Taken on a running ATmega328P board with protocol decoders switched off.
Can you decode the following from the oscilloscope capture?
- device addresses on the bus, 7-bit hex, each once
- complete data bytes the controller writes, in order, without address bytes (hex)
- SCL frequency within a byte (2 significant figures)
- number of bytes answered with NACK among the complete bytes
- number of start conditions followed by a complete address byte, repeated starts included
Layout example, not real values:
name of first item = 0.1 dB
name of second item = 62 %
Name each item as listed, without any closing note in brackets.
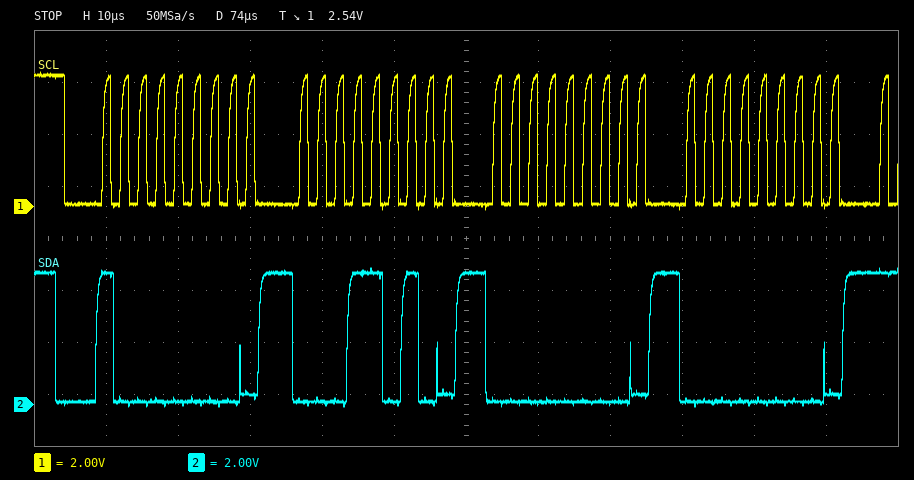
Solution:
device addresses on the bus, 7-bit hex, each once = 0x40
complete data bytes the controller writes, in order, without address bytes = 1A 00 00
SCL frequency within a byte = 400 kHz
number of bytes answered with NACK among the complete bytes = 0
number of start conditions followed by a complete address byte, repeated starts included = 1
